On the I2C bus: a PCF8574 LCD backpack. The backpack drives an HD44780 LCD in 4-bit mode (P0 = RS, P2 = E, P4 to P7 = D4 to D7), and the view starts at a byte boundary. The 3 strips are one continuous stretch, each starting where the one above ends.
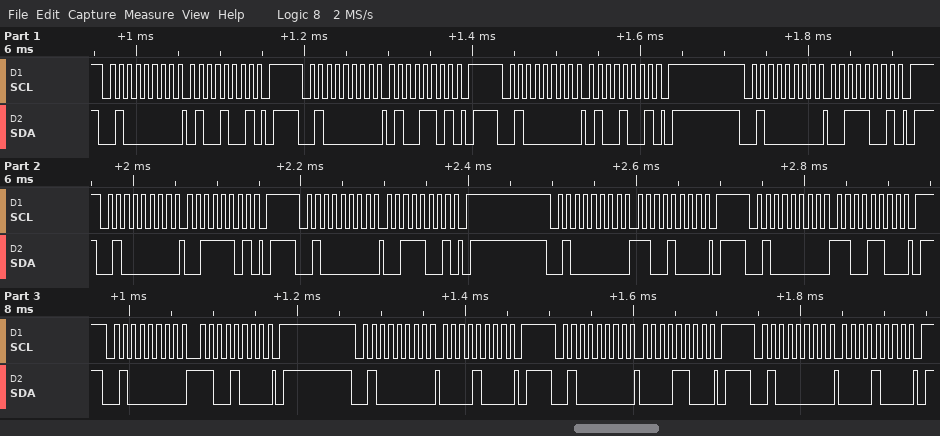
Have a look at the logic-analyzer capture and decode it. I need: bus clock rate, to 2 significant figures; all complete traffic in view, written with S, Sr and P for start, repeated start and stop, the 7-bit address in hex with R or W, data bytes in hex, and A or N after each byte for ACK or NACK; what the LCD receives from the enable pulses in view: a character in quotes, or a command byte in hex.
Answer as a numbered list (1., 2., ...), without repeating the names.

1. 100 kHz
2. S 20W A 49 A P S 20W A 4D A P S 20W A 49 A P S 20W A 39 A P S 20W A 3D A P S 20W A 39 A P S 20W A C8 A P S 20W A CC A P S 20W A C8 A P S 20W A 08 A P S 20W A 0C A P S 20W A 08 A P
3. 'C' 0xC0
